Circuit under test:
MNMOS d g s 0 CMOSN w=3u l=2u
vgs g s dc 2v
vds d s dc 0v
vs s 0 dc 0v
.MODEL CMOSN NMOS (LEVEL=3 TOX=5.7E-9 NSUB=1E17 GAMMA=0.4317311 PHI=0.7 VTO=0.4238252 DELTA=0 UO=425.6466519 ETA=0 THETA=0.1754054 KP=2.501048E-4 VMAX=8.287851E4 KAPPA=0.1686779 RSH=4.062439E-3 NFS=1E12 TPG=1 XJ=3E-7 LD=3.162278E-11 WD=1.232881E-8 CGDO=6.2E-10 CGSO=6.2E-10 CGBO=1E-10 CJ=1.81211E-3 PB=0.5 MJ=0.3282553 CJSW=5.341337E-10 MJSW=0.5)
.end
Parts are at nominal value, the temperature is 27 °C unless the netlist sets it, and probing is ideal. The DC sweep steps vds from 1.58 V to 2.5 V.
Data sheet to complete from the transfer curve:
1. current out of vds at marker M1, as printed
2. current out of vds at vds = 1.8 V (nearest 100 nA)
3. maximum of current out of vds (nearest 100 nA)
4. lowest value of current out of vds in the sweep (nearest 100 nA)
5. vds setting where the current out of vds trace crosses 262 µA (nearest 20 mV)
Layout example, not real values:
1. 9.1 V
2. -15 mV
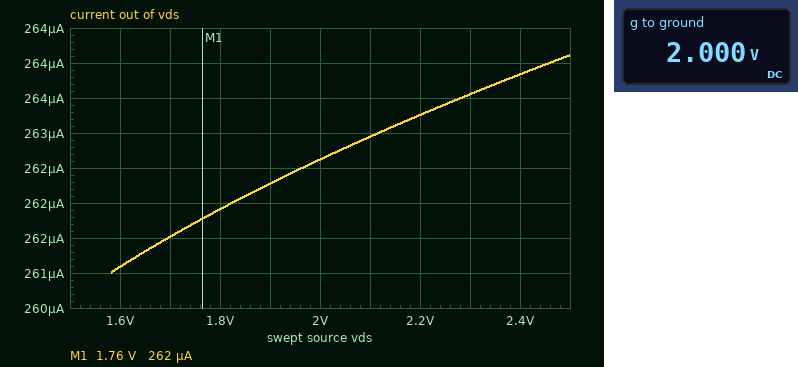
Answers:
1. 262 µA
2. 261.9 µA
3. 264.1 µA
4. 261.0 µA
5. 1.96 V
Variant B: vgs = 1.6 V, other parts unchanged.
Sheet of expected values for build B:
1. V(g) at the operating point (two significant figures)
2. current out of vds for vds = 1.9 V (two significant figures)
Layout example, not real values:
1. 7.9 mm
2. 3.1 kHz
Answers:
1. 1.6 V
2. 160 µA
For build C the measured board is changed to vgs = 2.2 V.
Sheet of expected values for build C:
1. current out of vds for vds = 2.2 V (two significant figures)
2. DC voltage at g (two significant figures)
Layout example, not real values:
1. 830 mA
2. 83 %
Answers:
1. 320 µA
2. 2.2 V
